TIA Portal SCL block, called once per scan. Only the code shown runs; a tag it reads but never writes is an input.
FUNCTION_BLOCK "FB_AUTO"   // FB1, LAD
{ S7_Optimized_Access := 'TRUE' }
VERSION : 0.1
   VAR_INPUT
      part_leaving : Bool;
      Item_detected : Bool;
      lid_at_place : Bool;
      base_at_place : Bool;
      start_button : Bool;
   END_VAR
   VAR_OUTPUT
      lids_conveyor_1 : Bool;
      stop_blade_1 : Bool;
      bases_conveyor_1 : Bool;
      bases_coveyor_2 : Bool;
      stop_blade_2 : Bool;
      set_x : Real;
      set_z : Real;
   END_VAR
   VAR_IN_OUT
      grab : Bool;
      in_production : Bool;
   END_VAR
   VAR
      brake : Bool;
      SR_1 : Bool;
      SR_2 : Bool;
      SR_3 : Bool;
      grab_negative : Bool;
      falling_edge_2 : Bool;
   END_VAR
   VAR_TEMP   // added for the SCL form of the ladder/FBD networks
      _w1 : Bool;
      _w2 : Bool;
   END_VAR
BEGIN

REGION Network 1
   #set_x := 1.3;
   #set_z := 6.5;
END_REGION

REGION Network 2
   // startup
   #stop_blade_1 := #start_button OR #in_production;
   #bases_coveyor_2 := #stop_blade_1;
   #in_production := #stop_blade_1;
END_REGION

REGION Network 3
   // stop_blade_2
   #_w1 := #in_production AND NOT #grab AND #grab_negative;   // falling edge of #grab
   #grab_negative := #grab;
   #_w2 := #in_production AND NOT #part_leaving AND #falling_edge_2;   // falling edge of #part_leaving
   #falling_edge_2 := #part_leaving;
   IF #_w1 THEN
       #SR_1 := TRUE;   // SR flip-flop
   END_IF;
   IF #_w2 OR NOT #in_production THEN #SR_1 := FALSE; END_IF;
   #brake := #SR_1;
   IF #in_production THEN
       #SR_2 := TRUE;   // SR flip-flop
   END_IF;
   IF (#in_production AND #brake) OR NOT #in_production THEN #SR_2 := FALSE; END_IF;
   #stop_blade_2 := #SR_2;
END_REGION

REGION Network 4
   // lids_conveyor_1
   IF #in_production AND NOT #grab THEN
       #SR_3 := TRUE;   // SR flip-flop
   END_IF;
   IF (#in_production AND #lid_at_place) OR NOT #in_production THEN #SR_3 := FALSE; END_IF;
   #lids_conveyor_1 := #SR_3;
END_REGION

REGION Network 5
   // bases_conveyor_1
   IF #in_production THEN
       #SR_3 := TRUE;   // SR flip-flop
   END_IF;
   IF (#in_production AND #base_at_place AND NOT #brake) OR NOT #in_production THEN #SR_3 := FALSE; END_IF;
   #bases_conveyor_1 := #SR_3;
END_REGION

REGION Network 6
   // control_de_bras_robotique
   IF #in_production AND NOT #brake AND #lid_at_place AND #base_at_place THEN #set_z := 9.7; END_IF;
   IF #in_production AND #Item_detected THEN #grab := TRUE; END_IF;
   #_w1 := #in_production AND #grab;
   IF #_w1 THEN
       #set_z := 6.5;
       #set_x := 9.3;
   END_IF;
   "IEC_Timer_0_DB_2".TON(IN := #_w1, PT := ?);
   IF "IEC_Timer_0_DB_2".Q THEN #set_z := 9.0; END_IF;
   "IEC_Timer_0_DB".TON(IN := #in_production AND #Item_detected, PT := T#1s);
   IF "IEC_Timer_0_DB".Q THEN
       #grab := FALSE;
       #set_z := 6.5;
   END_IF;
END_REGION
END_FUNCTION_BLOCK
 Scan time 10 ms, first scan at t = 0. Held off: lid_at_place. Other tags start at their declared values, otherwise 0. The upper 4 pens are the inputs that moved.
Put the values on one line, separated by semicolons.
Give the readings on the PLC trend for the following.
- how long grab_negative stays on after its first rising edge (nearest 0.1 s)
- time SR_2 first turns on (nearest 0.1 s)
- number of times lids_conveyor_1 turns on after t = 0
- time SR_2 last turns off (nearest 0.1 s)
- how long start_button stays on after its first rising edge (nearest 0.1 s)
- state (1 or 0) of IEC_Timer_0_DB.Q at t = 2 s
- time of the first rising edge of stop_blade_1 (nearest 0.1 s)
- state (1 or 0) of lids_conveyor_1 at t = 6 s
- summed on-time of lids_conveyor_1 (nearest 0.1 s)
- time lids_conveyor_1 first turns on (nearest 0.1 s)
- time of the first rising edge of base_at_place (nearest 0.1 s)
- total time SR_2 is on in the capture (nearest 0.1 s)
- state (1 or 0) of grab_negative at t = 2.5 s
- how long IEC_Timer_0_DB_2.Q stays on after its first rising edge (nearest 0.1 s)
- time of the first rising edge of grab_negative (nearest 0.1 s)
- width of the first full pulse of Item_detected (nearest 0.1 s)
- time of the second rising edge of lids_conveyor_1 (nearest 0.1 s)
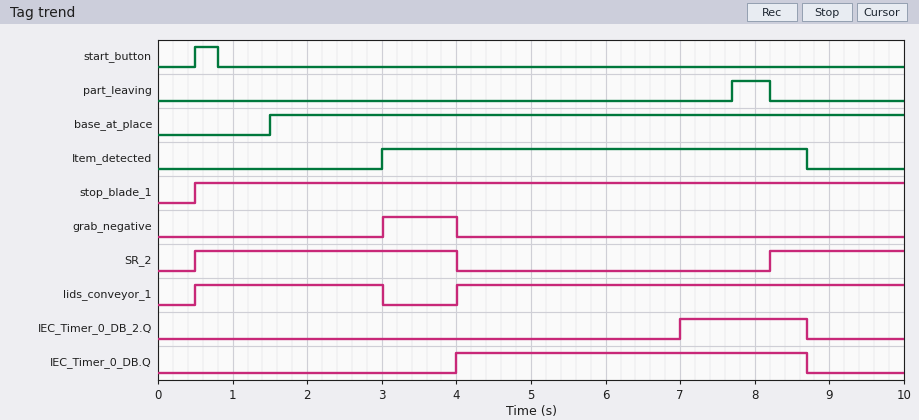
1.0 s; 0.5 s; 2; 4.0 s; 0.3 s; 0; 0.5 s; 1; 8.5 s; 0.5 s; 1.5 s; 5.3 s; 0; 1.7 s; 3.0 s; 5.7 s; 4.0 s
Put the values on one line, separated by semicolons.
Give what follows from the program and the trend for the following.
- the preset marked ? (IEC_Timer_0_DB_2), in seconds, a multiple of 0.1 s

4.0 s
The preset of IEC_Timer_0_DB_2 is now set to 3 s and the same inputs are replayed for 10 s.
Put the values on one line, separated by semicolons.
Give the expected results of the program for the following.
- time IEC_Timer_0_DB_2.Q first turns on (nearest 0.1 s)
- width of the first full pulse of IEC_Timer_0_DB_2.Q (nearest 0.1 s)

6.0 s; 2.7 s
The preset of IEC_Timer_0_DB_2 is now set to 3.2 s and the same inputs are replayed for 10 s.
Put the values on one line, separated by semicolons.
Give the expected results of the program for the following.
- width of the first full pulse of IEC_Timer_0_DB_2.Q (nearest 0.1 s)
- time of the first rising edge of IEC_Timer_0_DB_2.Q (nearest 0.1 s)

2.5 s; 6.2 s
